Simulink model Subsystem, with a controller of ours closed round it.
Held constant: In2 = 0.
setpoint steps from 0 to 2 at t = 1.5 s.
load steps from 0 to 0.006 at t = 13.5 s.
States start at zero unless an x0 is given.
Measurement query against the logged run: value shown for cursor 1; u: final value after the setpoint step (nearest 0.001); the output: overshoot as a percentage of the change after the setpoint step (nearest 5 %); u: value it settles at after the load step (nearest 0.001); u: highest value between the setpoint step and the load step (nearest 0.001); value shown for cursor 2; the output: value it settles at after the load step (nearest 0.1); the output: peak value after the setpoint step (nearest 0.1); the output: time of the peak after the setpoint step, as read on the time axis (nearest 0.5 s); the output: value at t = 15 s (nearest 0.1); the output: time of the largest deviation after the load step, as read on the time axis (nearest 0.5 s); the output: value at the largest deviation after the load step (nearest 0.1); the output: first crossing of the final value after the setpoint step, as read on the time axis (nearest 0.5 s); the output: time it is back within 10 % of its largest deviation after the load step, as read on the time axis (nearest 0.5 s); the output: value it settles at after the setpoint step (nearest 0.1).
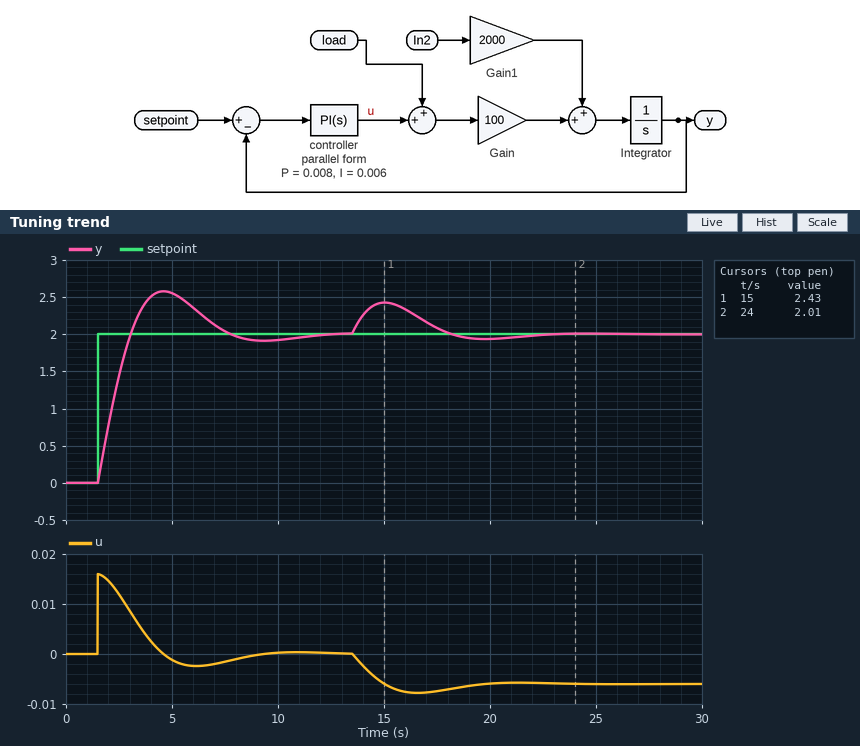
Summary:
2.43
0.000
30 %
-0.006
0.016
2.01
2.0
2.6
4.5 s
2.4
15.0 s
2.4
3.0 s
21.0 s
2.0
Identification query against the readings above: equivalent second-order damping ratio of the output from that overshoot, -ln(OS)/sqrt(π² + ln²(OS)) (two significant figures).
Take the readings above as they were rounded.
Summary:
0.36
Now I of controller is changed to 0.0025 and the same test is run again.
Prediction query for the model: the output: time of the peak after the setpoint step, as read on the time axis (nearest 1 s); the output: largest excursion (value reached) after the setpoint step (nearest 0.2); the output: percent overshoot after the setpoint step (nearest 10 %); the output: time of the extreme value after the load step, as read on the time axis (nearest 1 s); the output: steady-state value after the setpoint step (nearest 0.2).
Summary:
6 s
2.4
20 %
16 s
2.0
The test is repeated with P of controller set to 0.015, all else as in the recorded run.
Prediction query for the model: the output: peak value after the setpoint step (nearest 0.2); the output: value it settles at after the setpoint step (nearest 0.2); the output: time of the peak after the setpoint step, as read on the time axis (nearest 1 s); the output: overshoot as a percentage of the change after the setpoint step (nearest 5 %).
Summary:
2.2
2.0
4 s
15 %
